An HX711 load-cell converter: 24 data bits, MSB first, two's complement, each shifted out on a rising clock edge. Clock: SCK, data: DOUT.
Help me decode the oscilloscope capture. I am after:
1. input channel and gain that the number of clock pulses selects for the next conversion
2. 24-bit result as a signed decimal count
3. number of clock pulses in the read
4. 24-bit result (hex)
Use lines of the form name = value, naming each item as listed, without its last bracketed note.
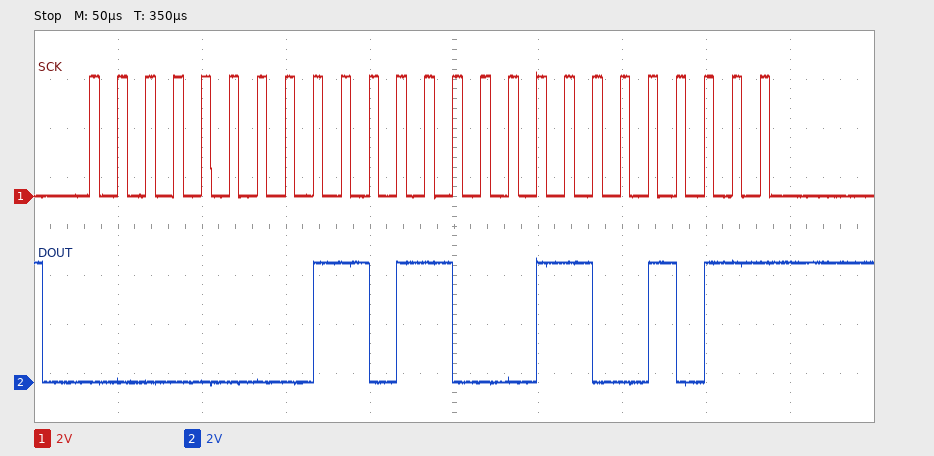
input channel and gain that the number of clock pulses selects for the next conversion = channel A, gain 128
24-bit result as a signed decimal count = 55499
number of clock pulses in the read = 25
24-bit result = 0x00D8CB
